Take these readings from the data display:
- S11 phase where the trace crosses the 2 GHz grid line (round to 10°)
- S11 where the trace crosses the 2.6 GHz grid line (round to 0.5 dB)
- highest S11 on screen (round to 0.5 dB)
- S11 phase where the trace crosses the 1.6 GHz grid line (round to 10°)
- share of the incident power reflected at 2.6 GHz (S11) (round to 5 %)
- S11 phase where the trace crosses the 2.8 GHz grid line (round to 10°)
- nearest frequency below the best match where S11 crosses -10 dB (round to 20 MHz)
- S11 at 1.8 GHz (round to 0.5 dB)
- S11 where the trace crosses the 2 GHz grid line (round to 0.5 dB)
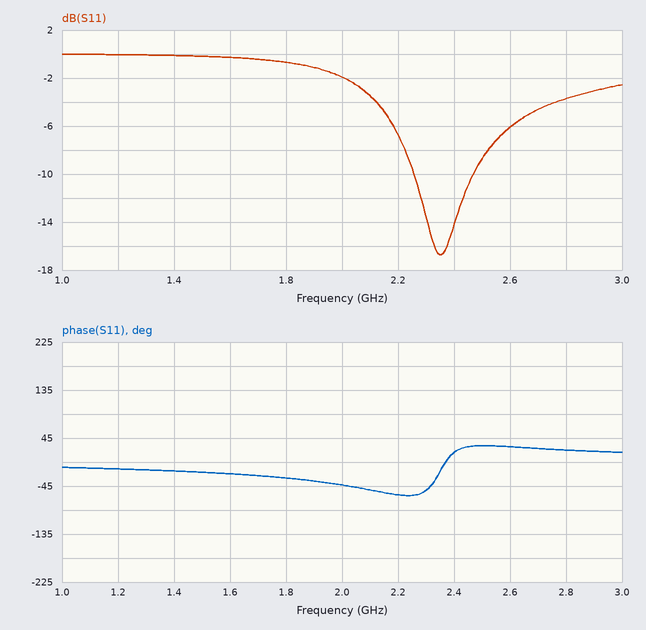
-40°
-6.0 dB
0.0 dB
-20°
25 %
20°
2.26 GHz
-0.5 dB
-2.0 dB
